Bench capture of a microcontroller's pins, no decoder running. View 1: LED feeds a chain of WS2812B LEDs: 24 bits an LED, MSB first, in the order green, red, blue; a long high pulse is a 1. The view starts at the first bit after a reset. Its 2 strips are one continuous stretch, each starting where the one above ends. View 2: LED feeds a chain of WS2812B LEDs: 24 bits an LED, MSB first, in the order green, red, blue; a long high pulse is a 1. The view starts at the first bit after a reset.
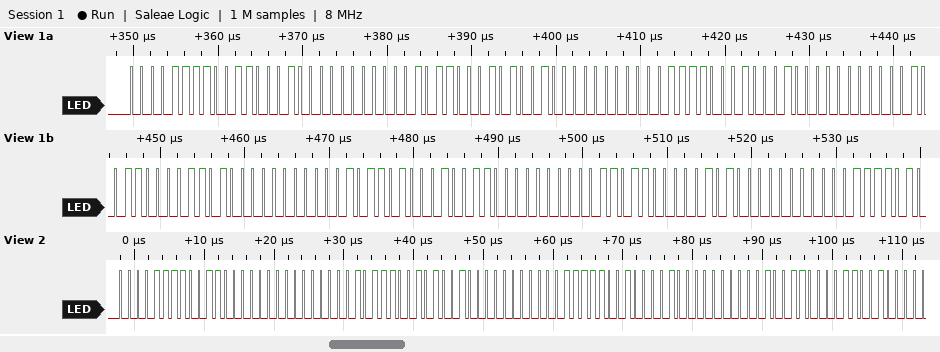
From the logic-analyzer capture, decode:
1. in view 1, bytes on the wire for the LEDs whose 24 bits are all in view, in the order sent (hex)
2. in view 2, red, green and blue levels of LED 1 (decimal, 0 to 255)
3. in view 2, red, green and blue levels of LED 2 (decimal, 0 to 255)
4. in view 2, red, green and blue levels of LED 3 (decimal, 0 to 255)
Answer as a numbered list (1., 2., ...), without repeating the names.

1. 0F 31 00 16 29 00 1E 22 00 26 1A 00 2D 13 00 36 0A 00
2. 48, 15, 0
3. 41, 23, 0
4. 33, 31, 0
